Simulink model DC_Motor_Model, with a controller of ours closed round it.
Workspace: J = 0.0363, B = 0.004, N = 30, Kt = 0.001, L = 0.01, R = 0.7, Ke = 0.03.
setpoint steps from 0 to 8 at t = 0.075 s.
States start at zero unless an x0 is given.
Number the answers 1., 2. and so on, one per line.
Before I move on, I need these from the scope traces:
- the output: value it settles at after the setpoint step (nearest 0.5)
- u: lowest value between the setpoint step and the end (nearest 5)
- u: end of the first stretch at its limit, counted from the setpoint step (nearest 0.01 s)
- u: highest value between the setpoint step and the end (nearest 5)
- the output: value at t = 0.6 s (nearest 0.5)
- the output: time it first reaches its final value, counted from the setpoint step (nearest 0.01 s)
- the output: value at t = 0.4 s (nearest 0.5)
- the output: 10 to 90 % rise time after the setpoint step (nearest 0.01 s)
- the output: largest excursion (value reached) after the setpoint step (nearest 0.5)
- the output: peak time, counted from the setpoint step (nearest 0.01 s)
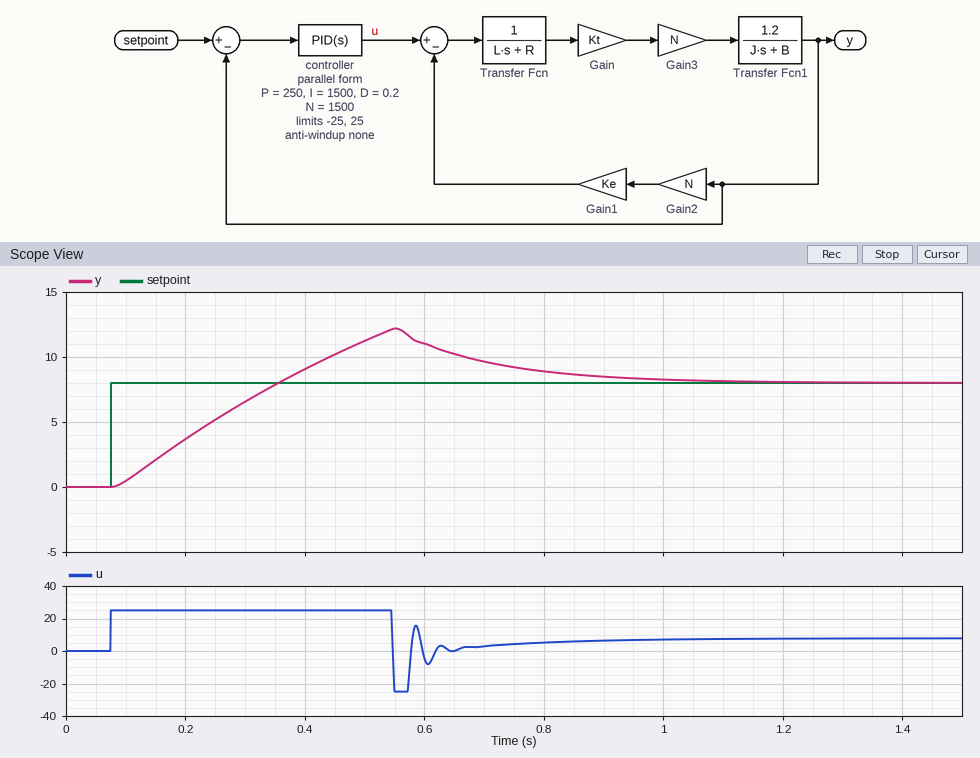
1. 8.0
2. -25
3. 0.47 s
4. 25
5. 11.0
6. 0.28 s
7. 9.0
8. 0.21 s
9. 12.0
10. 0.48 s
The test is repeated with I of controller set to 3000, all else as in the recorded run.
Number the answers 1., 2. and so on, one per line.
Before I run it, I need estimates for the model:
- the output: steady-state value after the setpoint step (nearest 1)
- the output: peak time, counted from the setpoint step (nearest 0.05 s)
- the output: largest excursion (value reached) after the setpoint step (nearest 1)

1. 8
2. 0.55 s
3. 13
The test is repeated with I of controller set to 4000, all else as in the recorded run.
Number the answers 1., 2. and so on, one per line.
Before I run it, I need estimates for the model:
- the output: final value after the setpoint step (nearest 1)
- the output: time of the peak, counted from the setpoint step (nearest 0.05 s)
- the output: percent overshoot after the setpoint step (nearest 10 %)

1. 8
2. 0.55 s
3. 70 %
